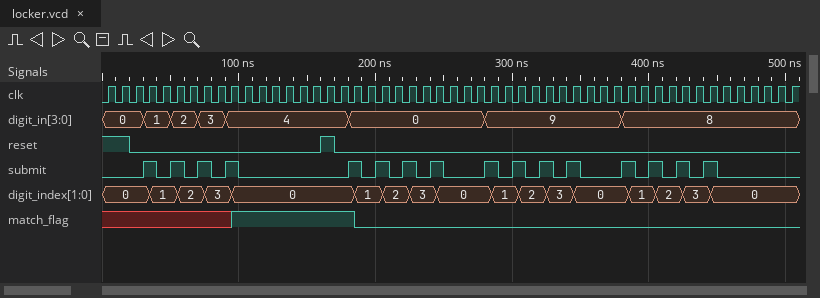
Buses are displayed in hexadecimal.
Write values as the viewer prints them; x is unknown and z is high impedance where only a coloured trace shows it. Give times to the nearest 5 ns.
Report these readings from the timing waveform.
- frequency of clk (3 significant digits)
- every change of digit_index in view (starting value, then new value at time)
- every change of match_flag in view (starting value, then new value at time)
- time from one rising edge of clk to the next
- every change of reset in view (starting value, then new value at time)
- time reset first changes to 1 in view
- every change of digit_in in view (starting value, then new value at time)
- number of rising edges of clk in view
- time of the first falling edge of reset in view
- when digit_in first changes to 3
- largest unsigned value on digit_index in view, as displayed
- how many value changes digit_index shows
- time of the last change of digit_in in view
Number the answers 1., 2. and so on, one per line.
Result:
1. 100 MHz
2. 0, 1 at 35 ns, 2 at 55 ns, 3 at 75 ns, 0 at 95 ns, 1 at 185 ns, 2 at 205 ns, 3 at 225 ns, 0 at 245 ns, 1 at 285 ns, 2 at 305 ns, 3 at 325 ns, 0 at 345 ns, 1 at 385 ns, 2 at 405 ns, 3 at 425 ns, 0 at 445 ns
3. x, 1 at 95 ns, 0 at 185 ns
4. 10 ns
5. 1, 0 at 20 ns, 1 at 160 ns, 0 at 170 ns
6. 160 ns
7. 0, 1 at 30 ns, 2 at 50 ns, 3 at 70 ns, 4 at 90 ns, 0 at 180 ns, 9 at 280 ns, 8 at 380 ns
8. 51
9. 20 ns
10. 70 ns
11. 3
12. 16
13. 380 ns
